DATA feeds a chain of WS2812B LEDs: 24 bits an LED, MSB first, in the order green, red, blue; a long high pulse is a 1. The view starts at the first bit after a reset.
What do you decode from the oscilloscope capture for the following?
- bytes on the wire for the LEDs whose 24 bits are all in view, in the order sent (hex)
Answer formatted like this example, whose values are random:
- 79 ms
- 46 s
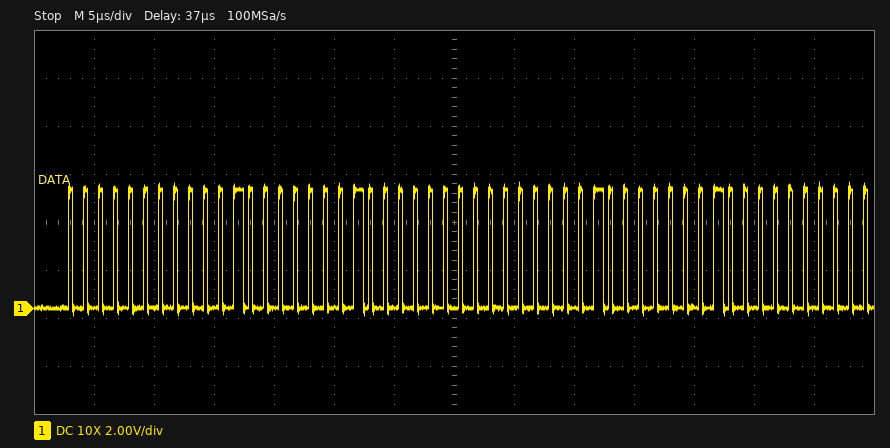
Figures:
- 00 10 10 00 10 10
